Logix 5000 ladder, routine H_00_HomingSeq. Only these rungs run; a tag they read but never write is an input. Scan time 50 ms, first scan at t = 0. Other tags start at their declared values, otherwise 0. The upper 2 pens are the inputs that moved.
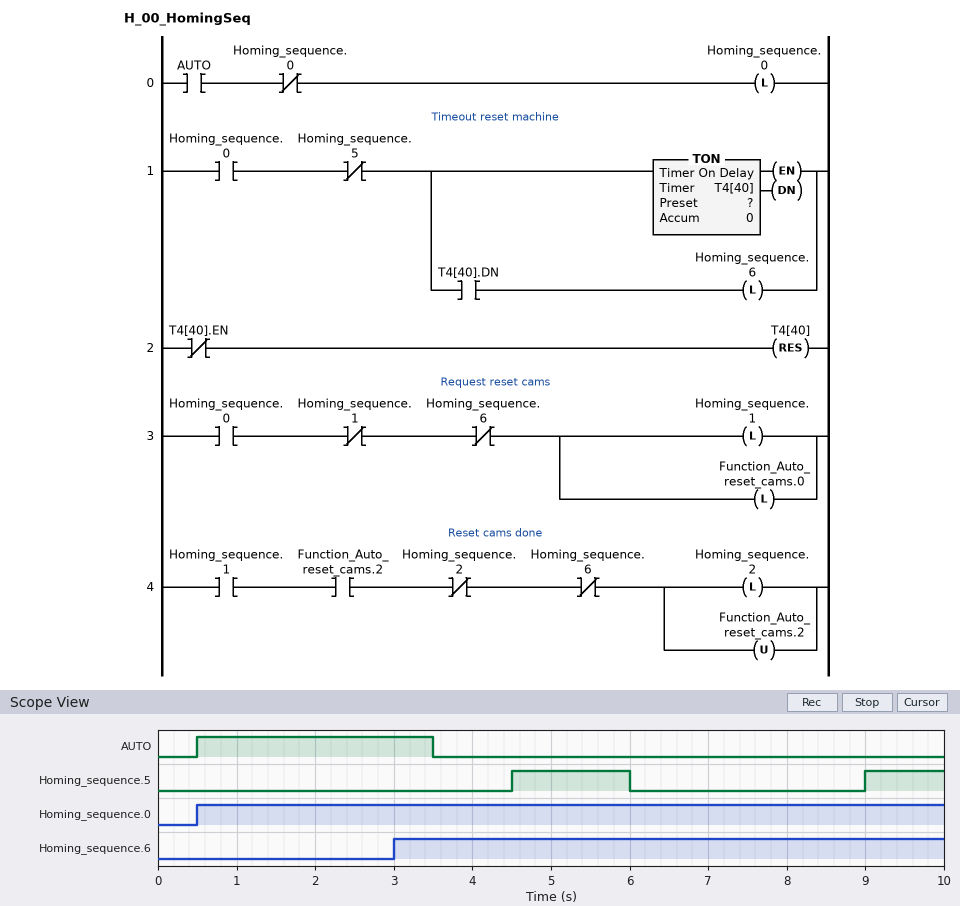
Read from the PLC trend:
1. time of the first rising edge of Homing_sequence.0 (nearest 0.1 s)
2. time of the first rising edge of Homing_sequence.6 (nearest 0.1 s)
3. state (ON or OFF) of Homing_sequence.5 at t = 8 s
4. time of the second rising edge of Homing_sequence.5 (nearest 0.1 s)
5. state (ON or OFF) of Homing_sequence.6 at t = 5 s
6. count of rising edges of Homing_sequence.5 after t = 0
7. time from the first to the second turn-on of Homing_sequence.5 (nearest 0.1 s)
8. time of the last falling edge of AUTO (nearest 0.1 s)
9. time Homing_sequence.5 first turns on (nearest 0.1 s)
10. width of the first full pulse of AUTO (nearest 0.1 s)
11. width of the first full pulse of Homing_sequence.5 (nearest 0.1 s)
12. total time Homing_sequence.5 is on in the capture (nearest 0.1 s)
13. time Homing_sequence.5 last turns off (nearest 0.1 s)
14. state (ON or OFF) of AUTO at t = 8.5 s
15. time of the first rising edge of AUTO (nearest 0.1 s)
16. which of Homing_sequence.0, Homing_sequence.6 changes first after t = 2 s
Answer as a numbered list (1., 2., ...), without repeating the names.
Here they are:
1. 0.5 s
2. 3.0 s
3. OFF
4. 9.0 s
5. ON
6. 2
7. 4.5 s
8. 3.5 s
9. 4.5 s
10. 3.0 s
11. 1.5 s
12. 2.5 s
13. 6.0 s
14. OFF
15. 0.5 s
16. Homing_sequence.6
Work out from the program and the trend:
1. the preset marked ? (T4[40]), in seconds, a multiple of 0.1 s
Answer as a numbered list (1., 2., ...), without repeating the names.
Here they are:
1. 2.5 s
